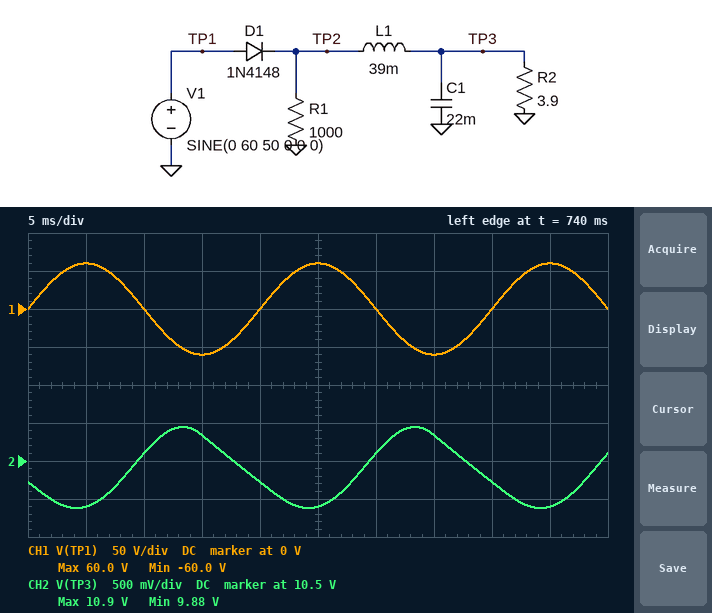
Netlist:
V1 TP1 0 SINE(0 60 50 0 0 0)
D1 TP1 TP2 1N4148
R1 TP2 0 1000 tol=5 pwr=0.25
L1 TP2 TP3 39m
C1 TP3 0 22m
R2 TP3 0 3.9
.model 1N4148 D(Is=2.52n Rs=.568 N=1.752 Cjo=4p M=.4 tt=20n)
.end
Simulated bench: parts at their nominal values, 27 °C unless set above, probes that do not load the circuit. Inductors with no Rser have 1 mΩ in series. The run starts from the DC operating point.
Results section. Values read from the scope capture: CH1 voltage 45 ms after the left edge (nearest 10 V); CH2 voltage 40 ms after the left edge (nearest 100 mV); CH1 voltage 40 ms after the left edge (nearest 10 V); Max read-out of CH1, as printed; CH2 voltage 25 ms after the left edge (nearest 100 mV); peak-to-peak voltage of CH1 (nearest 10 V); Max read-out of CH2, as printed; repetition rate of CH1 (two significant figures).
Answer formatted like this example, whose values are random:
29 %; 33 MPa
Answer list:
60 V; 10.2 V; 0 V; 60.0 V; 9.9 V; 120 V; 10.9 V; 50 Hz
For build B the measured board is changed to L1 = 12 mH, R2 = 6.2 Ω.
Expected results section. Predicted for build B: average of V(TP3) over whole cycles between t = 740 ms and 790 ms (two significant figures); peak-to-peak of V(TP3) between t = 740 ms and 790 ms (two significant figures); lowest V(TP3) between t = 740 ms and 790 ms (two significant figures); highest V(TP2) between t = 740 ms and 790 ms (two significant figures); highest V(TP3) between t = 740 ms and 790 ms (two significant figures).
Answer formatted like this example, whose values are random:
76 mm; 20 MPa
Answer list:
24 V; 1.9 V; 23 V; 55 V; 25 V
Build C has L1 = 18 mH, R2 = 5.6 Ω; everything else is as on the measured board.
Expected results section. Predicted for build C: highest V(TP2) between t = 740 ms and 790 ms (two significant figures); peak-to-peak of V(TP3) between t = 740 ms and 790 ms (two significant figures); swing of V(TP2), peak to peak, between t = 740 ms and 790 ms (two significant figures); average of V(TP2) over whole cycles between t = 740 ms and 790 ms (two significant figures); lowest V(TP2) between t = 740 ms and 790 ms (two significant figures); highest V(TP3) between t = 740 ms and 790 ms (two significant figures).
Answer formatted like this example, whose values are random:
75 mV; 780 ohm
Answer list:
56 V; 1.6 V; 110 V; 19 V; -51 V; 20 V
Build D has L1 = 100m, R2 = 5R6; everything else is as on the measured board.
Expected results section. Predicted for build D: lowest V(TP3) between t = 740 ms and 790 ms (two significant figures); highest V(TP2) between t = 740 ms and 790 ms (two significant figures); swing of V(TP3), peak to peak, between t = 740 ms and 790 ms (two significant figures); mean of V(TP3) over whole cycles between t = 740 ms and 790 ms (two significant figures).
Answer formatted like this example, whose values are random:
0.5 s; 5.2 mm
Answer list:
6.9 V; 58 V; 470 mV; 7.1 V
